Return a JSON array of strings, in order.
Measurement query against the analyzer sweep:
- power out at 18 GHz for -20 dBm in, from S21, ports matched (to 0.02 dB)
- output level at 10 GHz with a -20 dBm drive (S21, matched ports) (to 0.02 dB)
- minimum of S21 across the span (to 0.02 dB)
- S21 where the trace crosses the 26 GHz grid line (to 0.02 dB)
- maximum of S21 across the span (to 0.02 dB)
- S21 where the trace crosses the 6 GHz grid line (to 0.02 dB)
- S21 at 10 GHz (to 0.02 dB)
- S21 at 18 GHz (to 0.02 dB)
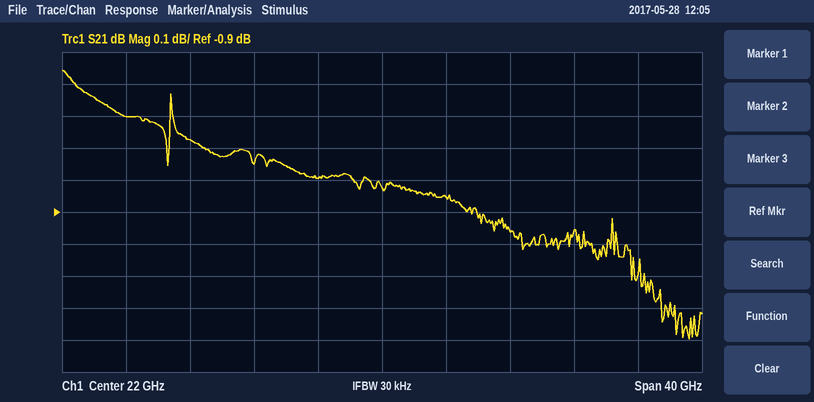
["-20.80 dBm", "-20.68 dBm", "-1.30 dB", "-0.86 dB", "-0.46 dB", "-0.60 dB", "-0.68 dB", "-0.80 dB"]
